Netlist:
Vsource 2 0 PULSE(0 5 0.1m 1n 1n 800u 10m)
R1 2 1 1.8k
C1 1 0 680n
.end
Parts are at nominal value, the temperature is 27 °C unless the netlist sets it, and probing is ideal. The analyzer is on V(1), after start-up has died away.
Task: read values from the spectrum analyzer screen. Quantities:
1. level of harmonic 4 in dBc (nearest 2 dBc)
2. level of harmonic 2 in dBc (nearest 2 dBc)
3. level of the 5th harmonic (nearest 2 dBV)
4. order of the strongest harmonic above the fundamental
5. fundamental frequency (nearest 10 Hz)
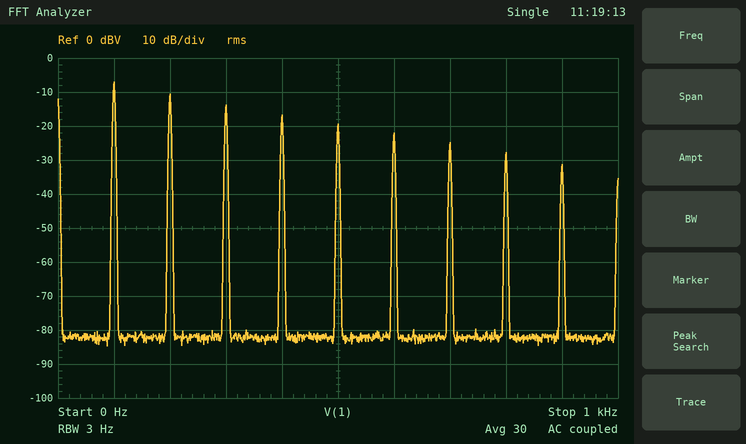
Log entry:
-10 dBc
-4 dBc
-20 dBV
2
100 Hz
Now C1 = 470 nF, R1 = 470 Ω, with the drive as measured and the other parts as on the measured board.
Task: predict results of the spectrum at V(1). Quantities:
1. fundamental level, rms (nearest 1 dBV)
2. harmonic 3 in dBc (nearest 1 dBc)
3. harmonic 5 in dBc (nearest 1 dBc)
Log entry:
-5 dBV
-1 dBc
-4 dBc
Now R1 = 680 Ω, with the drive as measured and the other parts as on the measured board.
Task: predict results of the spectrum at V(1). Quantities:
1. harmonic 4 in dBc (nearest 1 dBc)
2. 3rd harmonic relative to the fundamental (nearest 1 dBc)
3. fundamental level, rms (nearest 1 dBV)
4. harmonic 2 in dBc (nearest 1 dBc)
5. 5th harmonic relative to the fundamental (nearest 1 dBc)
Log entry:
-5 dBc
-3 dBc
-5 dBV
-1 dBc
-7 dBc
